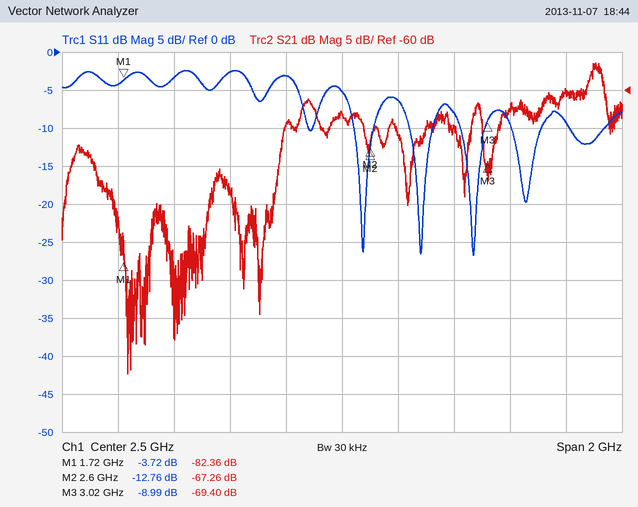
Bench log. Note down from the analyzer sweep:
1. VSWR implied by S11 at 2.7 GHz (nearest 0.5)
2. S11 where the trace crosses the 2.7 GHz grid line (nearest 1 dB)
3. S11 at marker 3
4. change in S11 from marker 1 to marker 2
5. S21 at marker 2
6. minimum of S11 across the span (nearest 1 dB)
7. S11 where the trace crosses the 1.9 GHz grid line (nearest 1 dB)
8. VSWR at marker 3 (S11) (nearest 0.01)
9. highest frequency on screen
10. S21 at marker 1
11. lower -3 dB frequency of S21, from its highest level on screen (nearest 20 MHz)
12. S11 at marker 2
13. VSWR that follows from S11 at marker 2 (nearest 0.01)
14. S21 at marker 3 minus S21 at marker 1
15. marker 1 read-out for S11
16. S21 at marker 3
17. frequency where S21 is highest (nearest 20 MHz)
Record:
3.0
-6 dB
-8.99 dB
-9.04 dB
-67.26 dB
-27 dB
-3 dB
2.10
3.5 GHz
-82.36 dB
3.38 GHz
-12.76 dB
1.60
12.96 dB
-3.72 dB
-69.40 dB
3.40 GHz
